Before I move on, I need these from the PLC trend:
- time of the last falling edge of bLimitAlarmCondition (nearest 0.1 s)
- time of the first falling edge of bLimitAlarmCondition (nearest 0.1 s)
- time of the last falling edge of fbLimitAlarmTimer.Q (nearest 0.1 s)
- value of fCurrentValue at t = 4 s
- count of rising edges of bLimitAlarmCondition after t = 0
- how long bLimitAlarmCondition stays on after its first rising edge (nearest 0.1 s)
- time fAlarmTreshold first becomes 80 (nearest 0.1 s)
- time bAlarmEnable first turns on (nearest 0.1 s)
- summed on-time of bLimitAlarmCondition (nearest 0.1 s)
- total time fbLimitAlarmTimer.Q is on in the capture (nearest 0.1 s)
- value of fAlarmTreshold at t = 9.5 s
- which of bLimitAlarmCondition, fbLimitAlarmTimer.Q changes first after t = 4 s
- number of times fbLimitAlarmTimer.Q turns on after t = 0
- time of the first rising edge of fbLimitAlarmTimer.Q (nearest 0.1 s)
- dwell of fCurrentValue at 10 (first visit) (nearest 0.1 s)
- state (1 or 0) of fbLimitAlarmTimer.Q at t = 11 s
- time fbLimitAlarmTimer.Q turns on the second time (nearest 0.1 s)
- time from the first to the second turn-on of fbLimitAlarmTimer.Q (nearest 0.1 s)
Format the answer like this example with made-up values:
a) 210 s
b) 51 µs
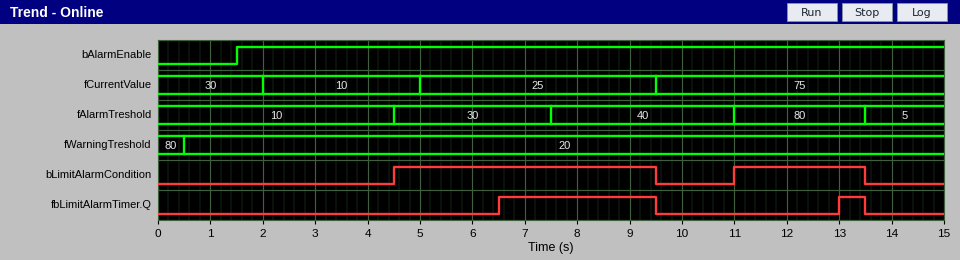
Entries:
a) 13.5 s
b) 9.5 s
c) 13.5 s
d) 10
e) 2
f) 5.0 s
g) 11.0 s
h) 1.5 s
i) 7.5 s
j) 3.5 s
k) 40
l) bLimitAlarmCondition
m) 2
n) 6.5 s
o) 3.0 s
p) 0
q) 13.0 s
r) 6.5 s
